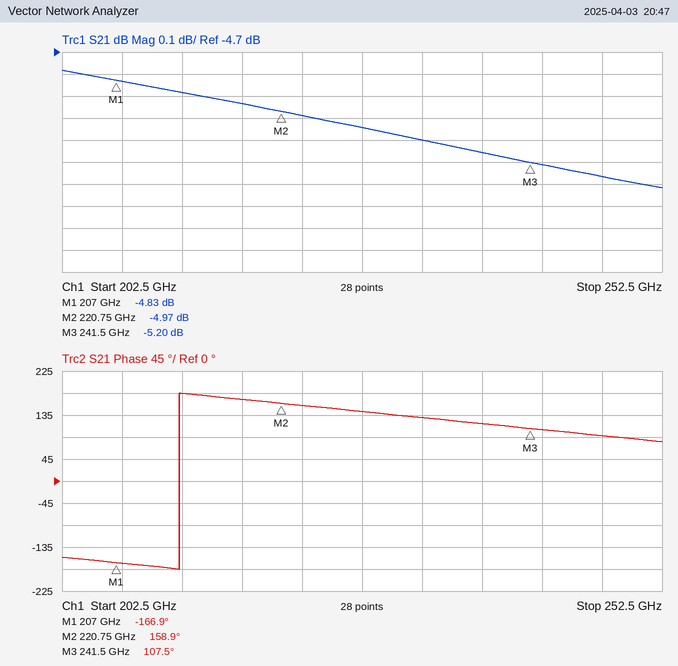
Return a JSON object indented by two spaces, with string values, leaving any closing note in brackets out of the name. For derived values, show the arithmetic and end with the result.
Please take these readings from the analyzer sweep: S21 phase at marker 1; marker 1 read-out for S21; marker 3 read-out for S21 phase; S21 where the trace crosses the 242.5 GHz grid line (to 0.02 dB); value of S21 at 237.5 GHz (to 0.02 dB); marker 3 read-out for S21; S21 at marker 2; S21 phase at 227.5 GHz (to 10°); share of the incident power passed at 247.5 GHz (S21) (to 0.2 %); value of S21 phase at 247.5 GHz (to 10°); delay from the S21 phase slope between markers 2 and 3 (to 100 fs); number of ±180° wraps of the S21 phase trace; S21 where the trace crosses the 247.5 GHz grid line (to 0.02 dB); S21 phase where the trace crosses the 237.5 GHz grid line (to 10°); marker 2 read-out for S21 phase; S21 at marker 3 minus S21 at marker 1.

{
  "S21 phase at marker 1": "-166.9°",
  "marker 1 read-out for S21": "-4.83 dB",
  "marker 3 read-out for S21 phase": "107.5°",
  "S21 where the trace crosses the 242.5 GHz grid line": "-5.22 dB",
  "value of S21 at 237.5 GHz": "-5.16 dB",
  "marker 3 read-out for S21": "-5.20 dB",
  "S21 at marker 2": "-4.97 dB",
  "S21 phase at 227.5 GHz": "140°",
  "share of the incident power passed at 247.5 GHz (S21)": "10^(-5.26/10) ≈ 29.8 %",
  "value of S21 phase at 247.5 GHz": "90°",
  "delay from the S21 phase slope between markers 2 and 3": "−(107.5° − (158.9°))/(360° × 20.75 GHz) ≈ 6.9 ps",
  "number of ±180° wraps of the S21 phase trace": "1",
  "S21 where the trace crosses the 247.5 GHz grid line": "-5.26 dB",
  "S21 phase where the trace crosses the 237.5 GHz grid line": "120°",
  "marker 2 read-out for S21 phase": "158.9°",
  "S21 at marker 3 minus S21 at marker 1": "-5.2 − (-4.83) = -0.37 dB"
}
